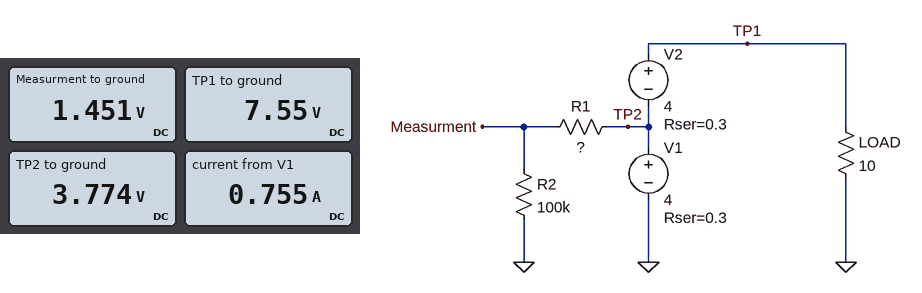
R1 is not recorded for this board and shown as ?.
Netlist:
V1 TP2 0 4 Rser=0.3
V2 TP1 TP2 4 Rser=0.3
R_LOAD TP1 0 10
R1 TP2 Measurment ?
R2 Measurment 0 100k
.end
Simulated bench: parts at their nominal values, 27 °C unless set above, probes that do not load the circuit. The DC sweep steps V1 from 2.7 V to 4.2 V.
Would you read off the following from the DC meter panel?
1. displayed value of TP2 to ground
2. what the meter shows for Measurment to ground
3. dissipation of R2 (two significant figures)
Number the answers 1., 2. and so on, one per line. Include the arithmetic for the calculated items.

1. 3.774 V
2. 1.451 V
3. (1.451 V)^2 / 100 kΩ = 21 µW
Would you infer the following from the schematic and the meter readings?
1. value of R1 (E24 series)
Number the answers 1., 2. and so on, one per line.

1. 160 kΩ
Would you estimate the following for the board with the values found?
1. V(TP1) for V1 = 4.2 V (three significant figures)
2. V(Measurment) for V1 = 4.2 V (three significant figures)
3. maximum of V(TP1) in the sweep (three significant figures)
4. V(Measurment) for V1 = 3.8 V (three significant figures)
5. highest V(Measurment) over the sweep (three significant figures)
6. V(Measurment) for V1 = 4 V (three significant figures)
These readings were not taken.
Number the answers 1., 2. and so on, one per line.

1. 7.74 V
2. 1.53 V
3. 7.74 V
4. 1.38 V
5. 1.53 V
6. 1.45 V
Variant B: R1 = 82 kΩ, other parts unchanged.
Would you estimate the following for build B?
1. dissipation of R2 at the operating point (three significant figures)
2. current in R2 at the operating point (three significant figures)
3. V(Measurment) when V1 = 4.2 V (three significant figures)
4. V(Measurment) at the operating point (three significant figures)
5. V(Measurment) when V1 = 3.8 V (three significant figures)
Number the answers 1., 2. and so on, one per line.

1. 43.0 µW
2. 20.7 µA
3. 2.18 V
4. 2.07 V
5. 1.97 V
